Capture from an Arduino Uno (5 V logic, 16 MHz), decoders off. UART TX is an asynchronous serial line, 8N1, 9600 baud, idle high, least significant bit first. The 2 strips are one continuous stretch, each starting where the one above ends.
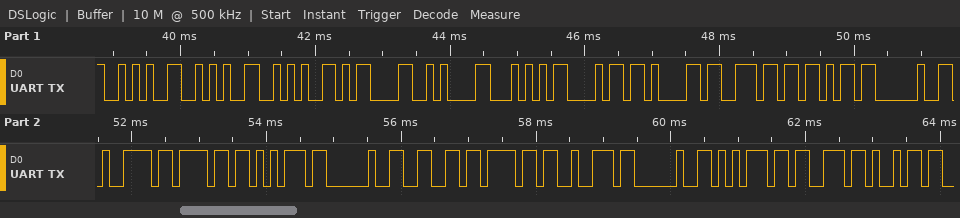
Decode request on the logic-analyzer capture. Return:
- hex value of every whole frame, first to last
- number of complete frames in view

2A 2A 2A 0D 0A 54 68 61 6E 6B 20 79 6F 75 20 66 6F 72 20 75 73 69
22
